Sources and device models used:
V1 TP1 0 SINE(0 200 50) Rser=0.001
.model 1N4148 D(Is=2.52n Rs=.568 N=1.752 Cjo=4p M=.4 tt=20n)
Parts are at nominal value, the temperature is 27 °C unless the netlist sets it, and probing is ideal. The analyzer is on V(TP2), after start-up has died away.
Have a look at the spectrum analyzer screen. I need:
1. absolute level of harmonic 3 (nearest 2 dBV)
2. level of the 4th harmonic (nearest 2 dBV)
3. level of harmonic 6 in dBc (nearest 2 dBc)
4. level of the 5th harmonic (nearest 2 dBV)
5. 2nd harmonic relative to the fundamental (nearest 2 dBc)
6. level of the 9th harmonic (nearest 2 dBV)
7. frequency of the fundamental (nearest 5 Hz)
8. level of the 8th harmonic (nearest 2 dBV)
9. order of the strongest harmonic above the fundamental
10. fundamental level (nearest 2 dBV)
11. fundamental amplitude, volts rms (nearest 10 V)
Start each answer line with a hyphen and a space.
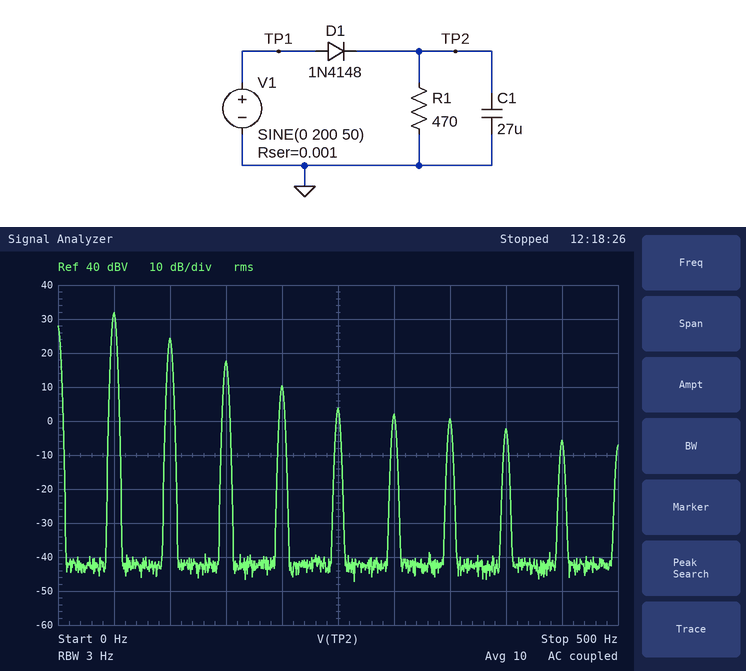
- 18 dBV
- 10 dBV
- -30 dBc
- 4 dBV
- -8 dBc
- -6 dBV
- 50 Hz
- -2 dBV
- 2
- 32 dBV
- 40 V
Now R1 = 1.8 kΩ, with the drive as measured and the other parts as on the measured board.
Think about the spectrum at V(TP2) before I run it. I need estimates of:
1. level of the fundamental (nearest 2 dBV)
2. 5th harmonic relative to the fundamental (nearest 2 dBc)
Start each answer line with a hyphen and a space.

- 24 dBV
- -18 dBc
